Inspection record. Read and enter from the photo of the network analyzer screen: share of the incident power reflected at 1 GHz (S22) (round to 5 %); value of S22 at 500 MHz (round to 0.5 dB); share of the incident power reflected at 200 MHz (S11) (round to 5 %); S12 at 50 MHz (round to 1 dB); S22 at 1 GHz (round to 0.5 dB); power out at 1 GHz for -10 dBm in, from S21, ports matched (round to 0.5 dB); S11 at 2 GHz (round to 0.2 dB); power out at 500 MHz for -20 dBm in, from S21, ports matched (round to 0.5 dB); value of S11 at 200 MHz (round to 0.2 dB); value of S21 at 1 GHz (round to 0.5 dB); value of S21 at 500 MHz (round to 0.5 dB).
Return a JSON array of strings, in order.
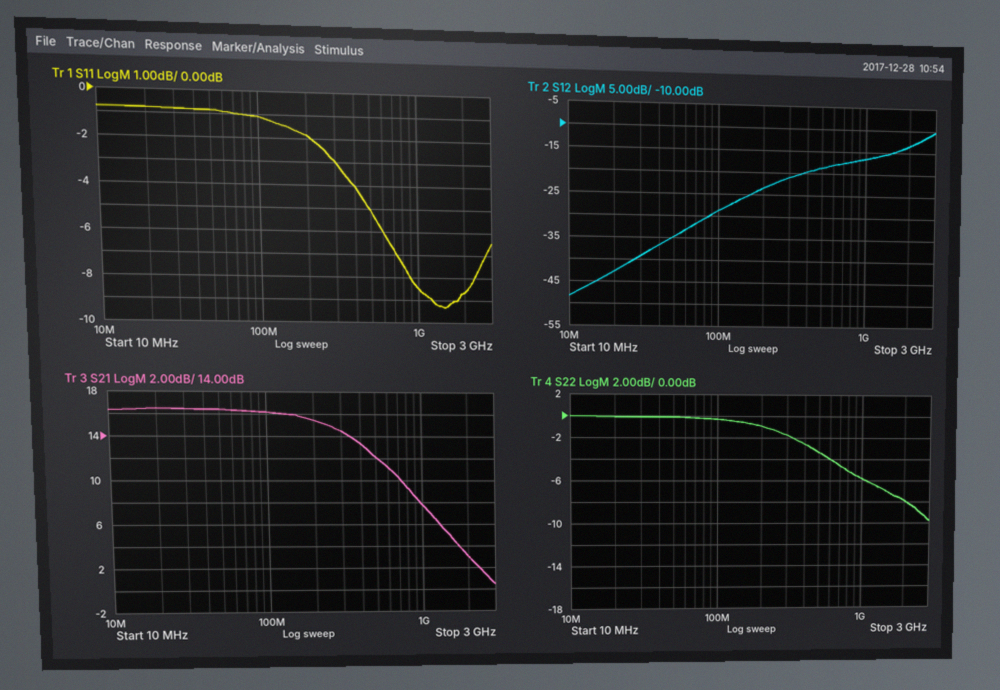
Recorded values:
["25 %", "-3.5 dB", "65 %", "-35 dB", "-6.0 dB", "-2.0 dBm", "-8.6 dB", "-8.0 dBm", "-1.8 dB", "8.0 dB", "12.0 dB"]
